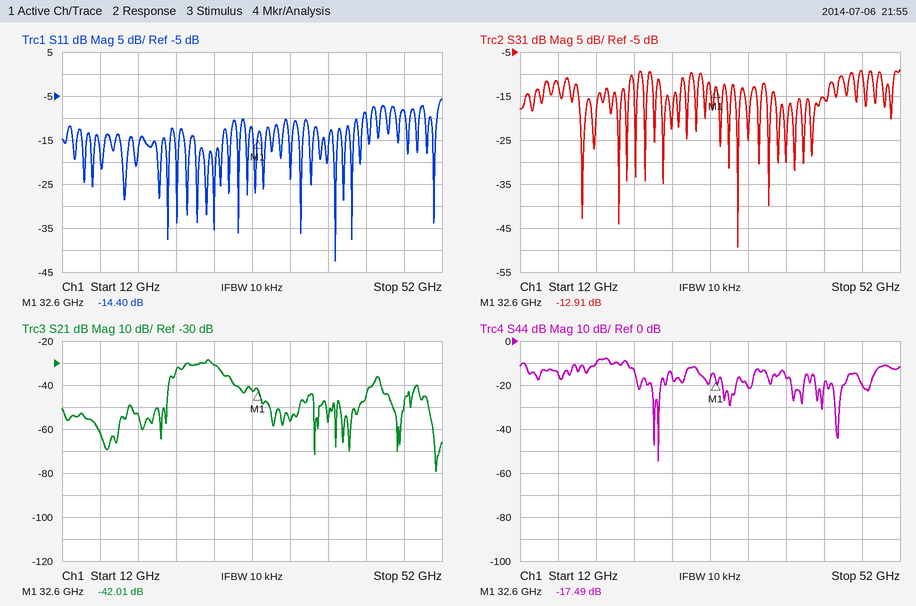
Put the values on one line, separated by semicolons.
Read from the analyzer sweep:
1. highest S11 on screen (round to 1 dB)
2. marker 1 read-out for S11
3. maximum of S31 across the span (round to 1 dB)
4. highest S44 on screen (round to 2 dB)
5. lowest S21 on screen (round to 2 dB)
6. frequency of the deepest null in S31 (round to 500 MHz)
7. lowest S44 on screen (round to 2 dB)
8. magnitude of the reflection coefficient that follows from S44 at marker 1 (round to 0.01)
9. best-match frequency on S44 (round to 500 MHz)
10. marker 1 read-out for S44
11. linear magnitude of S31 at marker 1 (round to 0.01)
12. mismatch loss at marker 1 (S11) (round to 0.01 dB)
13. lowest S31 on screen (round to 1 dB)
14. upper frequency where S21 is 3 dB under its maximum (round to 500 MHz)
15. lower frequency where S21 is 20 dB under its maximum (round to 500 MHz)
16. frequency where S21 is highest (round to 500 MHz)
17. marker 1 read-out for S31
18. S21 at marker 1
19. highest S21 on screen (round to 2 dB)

-6 dB; -14.40 dB; -9 dB; -8 dB; -80 dB; 35.0 GHz; -54 dB; 0.13; 26.5 GHz; -17.49 dB; 0.23; 0.16 dB; -49 dB; 28.5 GHz; 23.0 GHz; 27.5 GHz; -12.91 dB; -42.01 dB; -28 dB
